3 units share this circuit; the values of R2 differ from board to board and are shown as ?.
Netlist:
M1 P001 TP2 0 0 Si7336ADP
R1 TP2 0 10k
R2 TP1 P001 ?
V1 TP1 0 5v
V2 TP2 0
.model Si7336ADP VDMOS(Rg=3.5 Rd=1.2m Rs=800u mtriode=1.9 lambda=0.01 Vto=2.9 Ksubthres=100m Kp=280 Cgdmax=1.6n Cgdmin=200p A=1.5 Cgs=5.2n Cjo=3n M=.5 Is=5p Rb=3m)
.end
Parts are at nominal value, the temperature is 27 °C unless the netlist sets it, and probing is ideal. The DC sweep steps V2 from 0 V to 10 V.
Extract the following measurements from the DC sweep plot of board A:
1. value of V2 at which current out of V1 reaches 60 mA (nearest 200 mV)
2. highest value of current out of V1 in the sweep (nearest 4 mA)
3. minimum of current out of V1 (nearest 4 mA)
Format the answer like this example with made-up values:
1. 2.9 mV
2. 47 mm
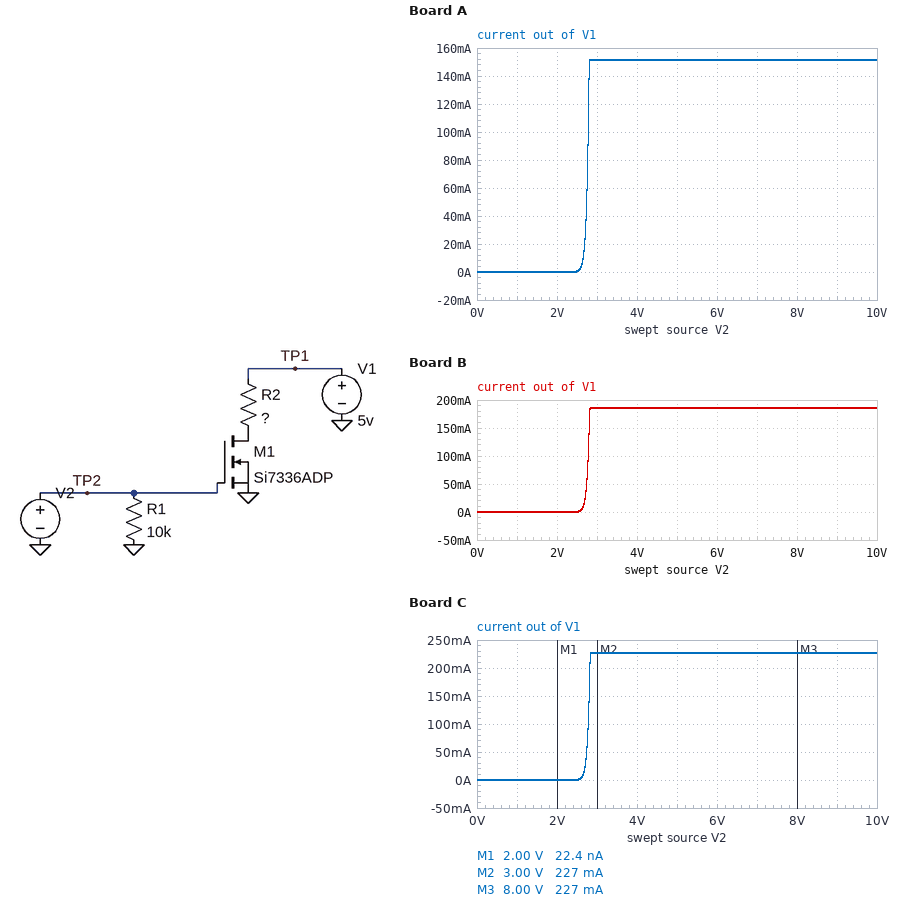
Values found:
1. 2.8 V
2. 152 mA
3. 0 A
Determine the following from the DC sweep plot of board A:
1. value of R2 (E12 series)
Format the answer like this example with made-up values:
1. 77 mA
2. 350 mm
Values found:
1. 33 Ω
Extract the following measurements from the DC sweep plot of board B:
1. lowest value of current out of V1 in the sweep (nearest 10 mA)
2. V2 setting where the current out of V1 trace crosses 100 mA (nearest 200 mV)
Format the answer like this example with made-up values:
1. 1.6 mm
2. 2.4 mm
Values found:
1. 0 A
2. 2.8 V
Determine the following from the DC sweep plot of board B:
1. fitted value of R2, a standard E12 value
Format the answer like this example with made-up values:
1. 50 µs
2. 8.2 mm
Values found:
1. 27 Ω
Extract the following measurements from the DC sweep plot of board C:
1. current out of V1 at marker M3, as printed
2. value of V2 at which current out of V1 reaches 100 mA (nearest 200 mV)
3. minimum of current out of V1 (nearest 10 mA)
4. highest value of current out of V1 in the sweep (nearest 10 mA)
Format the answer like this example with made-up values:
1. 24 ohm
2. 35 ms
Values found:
1. 227 mA
2. 2.8 V
3. 0 A
4. 230 mA
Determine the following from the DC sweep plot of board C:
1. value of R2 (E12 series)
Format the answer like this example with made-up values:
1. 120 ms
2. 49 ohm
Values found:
1. 22 Ω
